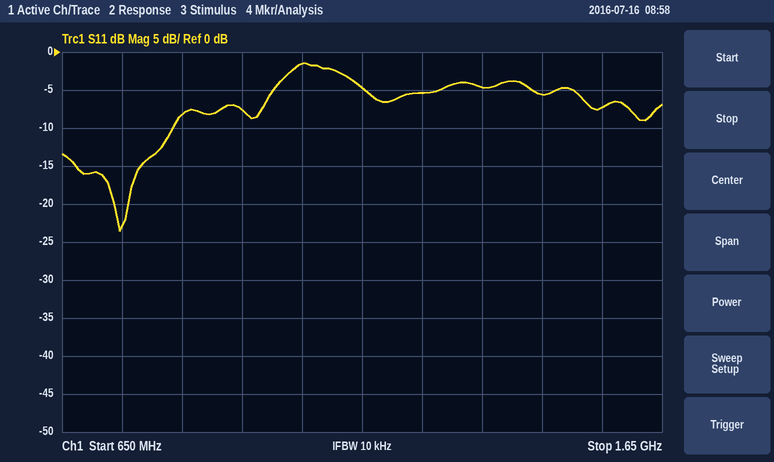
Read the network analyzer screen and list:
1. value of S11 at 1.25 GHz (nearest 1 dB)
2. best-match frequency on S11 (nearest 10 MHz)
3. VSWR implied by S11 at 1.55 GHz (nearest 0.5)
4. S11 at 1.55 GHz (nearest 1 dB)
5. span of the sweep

-5 dB
750 MHz
2.5
-7 dB
1 GHz
